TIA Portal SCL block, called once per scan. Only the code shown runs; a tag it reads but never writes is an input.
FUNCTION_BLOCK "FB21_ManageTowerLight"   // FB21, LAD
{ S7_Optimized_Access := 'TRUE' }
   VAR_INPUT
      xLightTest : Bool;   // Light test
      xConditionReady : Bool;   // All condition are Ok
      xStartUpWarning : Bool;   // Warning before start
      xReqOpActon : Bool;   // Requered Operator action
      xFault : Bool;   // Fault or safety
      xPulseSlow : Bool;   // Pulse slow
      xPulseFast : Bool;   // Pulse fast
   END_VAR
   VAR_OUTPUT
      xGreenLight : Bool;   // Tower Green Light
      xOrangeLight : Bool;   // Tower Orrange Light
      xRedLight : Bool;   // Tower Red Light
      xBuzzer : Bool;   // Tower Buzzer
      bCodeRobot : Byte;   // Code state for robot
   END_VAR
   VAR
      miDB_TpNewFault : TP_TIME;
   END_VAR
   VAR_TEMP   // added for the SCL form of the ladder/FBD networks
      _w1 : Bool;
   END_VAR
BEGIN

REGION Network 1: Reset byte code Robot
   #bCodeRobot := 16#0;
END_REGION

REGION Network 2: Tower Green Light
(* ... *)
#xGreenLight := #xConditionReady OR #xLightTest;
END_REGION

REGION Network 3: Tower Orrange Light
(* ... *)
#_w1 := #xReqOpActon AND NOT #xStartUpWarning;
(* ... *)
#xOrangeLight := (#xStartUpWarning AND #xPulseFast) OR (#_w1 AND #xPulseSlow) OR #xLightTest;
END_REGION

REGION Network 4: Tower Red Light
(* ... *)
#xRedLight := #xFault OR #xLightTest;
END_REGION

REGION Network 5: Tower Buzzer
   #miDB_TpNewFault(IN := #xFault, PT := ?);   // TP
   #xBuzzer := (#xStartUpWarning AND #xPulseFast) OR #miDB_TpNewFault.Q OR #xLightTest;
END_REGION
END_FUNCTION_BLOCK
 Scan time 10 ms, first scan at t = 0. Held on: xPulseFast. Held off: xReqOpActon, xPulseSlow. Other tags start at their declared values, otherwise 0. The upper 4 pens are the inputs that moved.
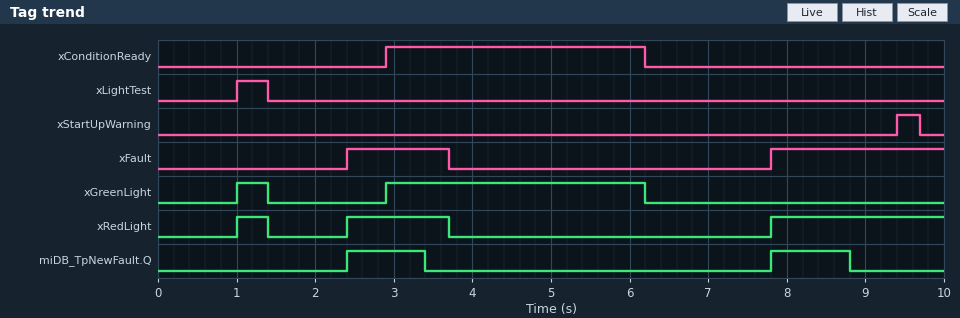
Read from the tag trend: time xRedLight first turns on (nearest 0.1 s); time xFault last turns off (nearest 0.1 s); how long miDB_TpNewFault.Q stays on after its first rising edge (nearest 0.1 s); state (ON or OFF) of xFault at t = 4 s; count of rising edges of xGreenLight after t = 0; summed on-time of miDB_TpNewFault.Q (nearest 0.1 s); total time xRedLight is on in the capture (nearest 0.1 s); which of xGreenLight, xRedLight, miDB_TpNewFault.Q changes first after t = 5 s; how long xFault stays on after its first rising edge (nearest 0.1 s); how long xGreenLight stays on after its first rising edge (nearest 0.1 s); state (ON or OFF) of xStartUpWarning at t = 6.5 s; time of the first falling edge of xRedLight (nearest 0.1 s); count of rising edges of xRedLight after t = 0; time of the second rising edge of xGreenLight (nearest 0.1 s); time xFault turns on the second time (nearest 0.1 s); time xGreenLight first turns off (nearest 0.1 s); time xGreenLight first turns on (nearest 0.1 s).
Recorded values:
1.0 s
3.7 s
1.0 s
OFF
2
2.0 s
3.9 s
xGreenLight
1.3 s
0.4 s
OFF
1.4 s
3
2.9 s
7.8 s
1.4 s
1.0 s
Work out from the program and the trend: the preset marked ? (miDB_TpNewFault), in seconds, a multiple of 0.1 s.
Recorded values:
1.0 s
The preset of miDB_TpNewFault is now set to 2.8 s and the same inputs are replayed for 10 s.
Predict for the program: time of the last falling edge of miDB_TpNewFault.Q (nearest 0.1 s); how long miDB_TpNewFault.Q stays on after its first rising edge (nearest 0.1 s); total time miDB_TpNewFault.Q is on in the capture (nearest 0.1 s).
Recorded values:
5.2 s
2.8 s
5.0 s
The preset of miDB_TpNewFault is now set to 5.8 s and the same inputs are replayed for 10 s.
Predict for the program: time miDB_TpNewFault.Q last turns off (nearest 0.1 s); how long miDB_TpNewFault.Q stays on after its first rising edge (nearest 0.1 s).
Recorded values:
8.2 s
5.8 s
